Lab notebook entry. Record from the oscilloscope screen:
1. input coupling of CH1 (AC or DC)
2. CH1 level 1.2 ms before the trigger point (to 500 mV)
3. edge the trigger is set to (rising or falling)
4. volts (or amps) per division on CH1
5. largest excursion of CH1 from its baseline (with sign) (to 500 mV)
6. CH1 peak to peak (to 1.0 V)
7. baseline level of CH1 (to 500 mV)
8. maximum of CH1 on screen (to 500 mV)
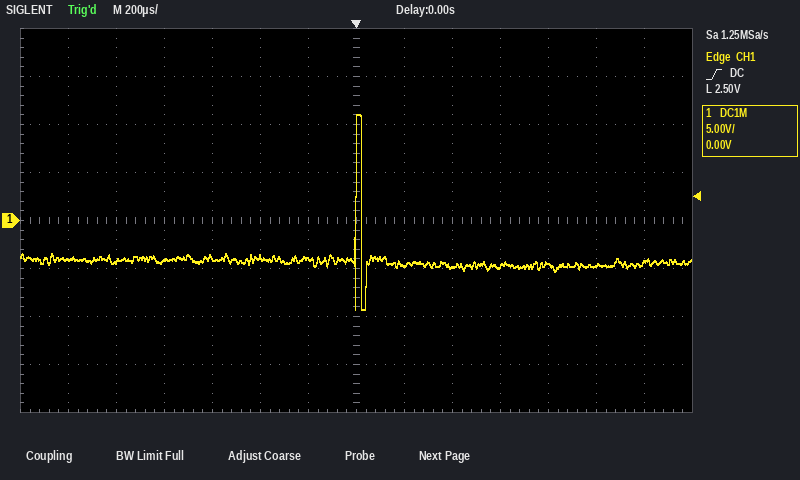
DC
-4.0 V
rising
5 V
+15.5 V
20.0 V
-4.5 V
11.0 V
